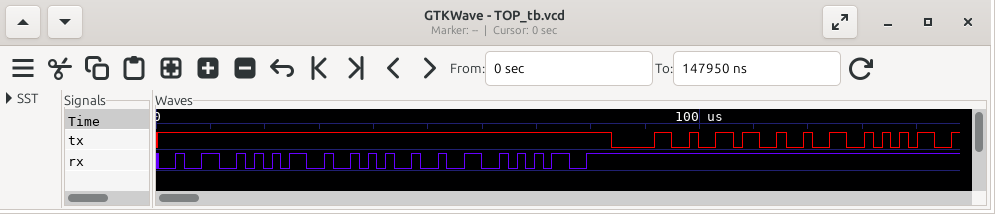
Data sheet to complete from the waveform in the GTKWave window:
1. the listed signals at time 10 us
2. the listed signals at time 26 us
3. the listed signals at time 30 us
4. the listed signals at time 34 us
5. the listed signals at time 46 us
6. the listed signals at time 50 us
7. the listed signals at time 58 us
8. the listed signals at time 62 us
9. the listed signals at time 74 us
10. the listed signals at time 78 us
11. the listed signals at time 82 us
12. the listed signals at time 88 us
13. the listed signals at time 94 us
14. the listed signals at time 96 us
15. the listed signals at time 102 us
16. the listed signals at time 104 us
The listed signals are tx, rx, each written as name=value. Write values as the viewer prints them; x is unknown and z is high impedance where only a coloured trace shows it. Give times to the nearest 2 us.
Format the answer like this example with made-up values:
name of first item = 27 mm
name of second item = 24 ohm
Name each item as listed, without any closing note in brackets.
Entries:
the listed signals at time 10 us = tx=1, rx=1
the listed signals at time 26 us = tx=1, rx=1
the listed signals at time 30 us = tx=1, rx=0
the listed signals at time 34 us = tx=1, rx=0
the listed signals at time 46 us = tx=1, rx=0
the listed signals at time 50 us = tx=1, rx=0
the listed signals at time 58 us = tx=1, rx=1
the listed signals at time 62 us = tx=1, rx=0
the listed signals at time 74 us = tx=1, rx=1
the listed signals at time 78 us = tx=1, rx=0
the listed signals at time 82 us = tx=1, rx=1
the listed signals at time 88 us = tx=0, rx=1
the listed signals at time 94 us = tx=1, rx=1
the listed signals at time 96 us = tx=0, rx=1
the listed signals at time 102 us = tx=0, rx=1
the listed signals at time 104 us = tx=1, rx=1
